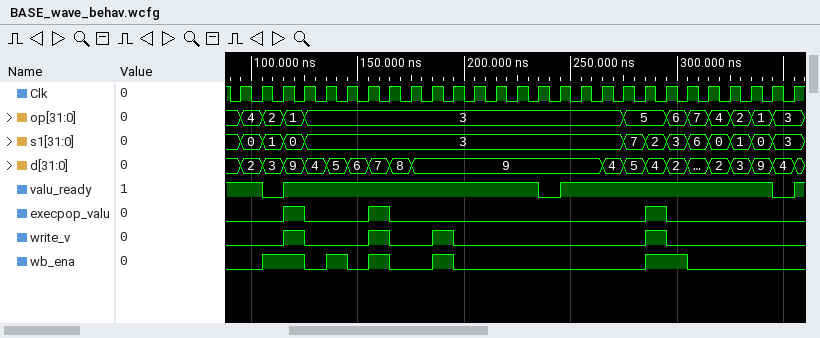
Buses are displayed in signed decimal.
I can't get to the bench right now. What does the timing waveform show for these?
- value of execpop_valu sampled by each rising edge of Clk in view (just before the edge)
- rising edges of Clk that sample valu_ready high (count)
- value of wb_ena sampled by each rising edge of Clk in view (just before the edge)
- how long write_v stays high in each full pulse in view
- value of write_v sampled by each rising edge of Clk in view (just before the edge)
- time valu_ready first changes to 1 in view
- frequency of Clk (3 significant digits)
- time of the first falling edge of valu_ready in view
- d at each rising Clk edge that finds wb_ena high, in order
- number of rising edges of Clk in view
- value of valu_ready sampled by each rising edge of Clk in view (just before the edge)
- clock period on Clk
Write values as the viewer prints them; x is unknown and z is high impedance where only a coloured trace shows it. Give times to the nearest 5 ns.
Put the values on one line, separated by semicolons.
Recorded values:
0 0 0 1 0 0 0 1 0 0 0 0 0 0 0 0 0 0 0 0 1 0 0 0 0 0 0; 24; 0 0 1 1 0 1 0 1 0 0 1 0 0 0 0 0 0 0 0 0 1 1 0 0 0 0 0; 10 ns, 10 ns, 10 ns, 10 ns; 0 0 0 1 0 0 0 1 0 0 1 0 0 0 0 0 0 0 0 0 1 0 0 0 0 0 0; 115 ns; 100 MHz; 105 ns; 3, 9, 5, 7, 9, 4, 2; 27; 1 1 0 1 1 1 1 1 1 1 1 1 1 1 1 0 1 1 1 1 1 1 1 1 1 1 0; 10 ns
